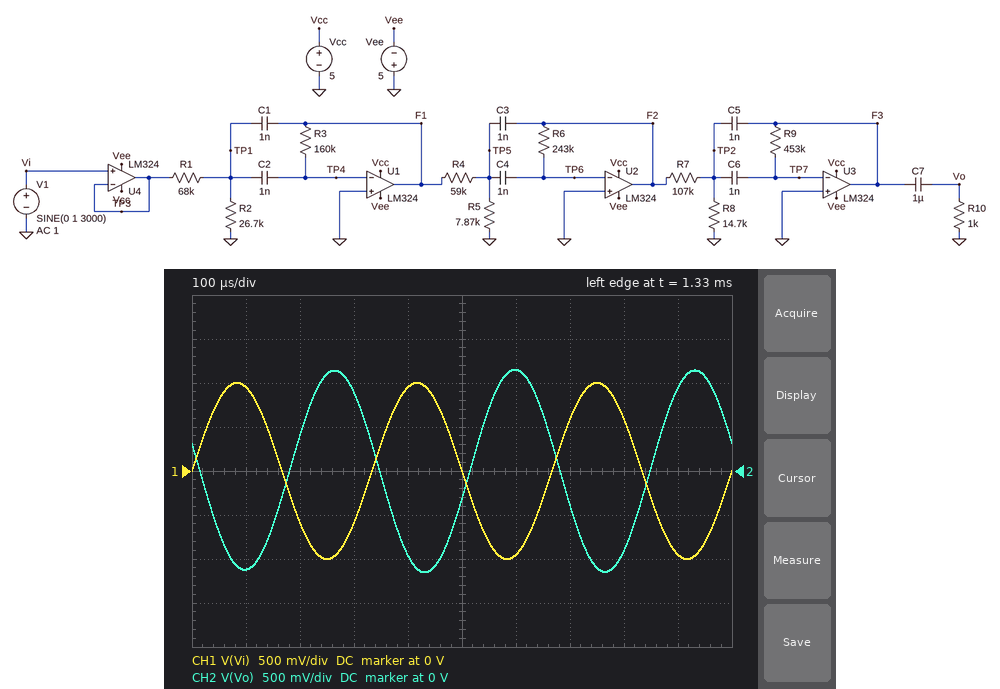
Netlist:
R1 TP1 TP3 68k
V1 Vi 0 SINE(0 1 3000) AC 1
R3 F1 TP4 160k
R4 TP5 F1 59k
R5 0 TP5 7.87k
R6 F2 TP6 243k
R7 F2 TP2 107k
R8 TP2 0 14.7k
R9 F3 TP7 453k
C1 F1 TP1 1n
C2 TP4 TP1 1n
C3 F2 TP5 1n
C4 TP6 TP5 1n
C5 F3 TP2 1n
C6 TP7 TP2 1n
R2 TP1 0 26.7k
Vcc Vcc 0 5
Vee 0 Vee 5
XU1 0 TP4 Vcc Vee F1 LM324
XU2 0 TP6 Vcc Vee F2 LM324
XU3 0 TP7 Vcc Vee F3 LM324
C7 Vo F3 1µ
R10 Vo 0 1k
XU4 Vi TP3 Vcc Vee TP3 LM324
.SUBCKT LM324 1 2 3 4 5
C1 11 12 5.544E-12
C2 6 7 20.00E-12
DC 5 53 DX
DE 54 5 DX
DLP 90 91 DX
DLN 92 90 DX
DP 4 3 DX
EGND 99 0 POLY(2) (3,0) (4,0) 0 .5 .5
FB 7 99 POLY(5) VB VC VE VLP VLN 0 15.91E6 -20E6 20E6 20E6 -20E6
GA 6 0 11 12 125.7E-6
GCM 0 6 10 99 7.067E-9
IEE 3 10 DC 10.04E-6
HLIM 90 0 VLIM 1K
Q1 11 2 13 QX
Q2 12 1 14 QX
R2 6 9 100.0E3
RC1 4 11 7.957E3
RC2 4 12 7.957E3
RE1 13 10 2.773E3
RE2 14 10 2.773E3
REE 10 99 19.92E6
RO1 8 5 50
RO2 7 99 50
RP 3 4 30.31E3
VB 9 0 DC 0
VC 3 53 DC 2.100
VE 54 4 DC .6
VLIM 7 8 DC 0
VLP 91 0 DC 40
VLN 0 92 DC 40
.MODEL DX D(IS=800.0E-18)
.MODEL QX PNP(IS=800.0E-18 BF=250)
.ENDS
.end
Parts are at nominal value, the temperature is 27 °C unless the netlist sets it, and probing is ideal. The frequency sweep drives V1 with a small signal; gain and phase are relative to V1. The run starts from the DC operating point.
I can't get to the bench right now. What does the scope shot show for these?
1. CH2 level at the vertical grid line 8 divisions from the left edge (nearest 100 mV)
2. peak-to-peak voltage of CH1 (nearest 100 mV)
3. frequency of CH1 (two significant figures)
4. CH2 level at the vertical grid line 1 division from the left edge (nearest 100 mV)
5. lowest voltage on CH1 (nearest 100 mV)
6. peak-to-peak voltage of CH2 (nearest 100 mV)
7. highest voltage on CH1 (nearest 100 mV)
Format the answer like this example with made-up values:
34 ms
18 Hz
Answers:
-900 mV
2.0 V
3.0 kHz
-1.1 V
-1.0 V
2.3 V
1.0 V
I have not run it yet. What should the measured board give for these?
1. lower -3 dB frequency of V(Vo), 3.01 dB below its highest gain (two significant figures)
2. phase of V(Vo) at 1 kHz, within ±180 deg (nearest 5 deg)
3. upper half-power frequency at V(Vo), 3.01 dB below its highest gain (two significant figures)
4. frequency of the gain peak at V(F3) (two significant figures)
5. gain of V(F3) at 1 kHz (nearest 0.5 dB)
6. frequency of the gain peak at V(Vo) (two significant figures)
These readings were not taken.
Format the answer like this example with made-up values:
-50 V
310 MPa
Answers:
2.0 kHz
65 deg
4.0 kHz
3.2 kHz
-31.5 dB
3.2 kHz
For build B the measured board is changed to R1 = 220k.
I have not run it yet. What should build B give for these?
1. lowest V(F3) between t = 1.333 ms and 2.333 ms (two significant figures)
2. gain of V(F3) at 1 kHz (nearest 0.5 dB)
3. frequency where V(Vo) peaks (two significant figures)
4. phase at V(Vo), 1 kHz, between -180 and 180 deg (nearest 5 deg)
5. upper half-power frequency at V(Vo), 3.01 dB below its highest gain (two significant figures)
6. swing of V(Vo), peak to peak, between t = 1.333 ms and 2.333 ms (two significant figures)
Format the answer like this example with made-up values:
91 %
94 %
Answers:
-340 mV
-40.0 dB
2.3 kHz
60 deg
3.8 kHz
670 mV
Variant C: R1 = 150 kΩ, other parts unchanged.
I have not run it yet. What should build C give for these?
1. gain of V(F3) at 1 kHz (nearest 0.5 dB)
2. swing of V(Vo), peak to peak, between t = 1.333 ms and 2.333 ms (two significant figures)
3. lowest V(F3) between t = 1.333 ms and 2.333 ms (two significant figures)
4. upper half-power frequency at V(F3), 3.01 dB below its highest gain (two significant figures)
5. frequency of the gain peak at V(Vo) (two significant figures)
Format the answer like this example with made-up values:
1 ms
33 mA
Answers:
-37.0 dB
1.0 V
-510 mV
3.9 kHz
2.3 kHz
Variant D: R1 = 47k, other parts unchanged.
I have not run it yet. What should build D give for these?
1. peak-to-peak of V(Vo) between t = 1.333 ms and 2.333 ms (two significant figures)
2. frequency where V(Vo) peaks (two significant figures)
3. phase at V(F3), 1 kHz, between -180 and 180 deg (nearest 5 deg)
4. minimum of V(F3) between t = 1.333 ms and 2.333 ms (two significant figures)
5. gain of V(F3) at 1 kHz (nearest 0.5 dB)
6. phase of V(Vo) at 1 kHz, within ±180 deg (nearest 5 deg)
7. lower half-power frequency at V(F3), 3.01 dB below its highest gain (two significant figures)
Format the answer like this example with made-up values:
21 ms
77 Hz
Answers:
3.4 V
3.4 kHz
60 deg
-1.7 V
-29.5 dB
70 deg
2.1 kHz
